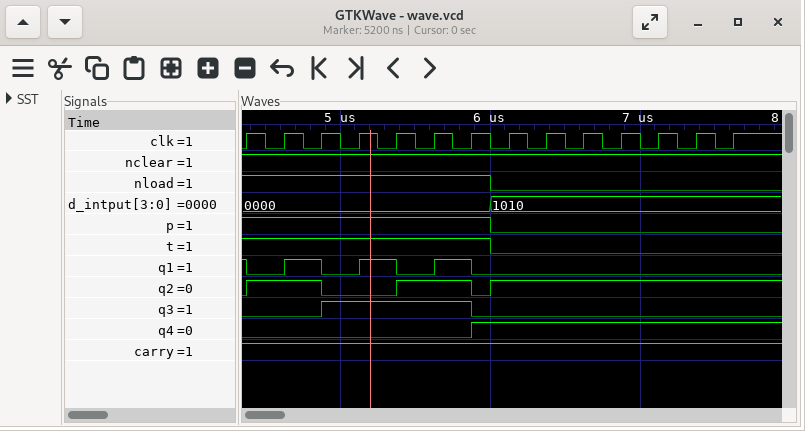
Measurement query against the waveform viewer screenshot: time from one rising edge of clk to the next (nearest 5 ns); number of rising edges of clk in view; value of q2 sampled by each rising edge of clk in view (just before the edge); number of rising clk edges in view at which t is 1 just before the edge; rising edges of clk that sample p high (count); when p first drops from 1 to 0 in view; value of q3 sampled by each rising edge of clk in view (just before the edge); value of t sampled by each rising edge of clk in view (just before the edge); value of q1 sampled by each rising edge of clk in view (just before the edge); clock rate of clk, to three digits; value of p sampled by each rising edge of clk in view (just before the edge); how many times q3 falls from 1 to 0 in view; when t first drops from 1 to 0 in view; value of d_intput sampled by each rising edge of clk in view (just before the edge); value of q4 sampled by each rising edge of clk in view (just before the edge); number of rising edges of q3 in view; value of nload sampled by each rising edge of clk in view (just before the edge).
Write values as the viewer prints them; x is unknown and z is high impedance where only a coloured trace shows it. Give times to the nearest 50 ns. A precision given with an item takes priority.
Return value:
250 ns
14
0 1 1 0 0 1 1 1 1 1 1 1 1 1
7
7
6000 ns
0 0 0 1 1 1 1 0 0 0 0 0 0 0
1 1 1 1 1 1 1 0 0 0 0 0 0 0
1 0 1 0 1 0 1 0 0 0 0 0 0 0
4.00 MHz
1 1 1 1 1 1 1 0 0 0 0 0 0 0
1
6000 ns
0000, 0000, 0000, 0000, 0000, 0000, 0000, 1010, 1010, 1010, 1010, 1010, 1010, 1010
0 0 0 0 0 0 0 1 1 1 1 1 1 1
1
1 1 1 1 1 1 1 0 0 0 0 0 0 0
